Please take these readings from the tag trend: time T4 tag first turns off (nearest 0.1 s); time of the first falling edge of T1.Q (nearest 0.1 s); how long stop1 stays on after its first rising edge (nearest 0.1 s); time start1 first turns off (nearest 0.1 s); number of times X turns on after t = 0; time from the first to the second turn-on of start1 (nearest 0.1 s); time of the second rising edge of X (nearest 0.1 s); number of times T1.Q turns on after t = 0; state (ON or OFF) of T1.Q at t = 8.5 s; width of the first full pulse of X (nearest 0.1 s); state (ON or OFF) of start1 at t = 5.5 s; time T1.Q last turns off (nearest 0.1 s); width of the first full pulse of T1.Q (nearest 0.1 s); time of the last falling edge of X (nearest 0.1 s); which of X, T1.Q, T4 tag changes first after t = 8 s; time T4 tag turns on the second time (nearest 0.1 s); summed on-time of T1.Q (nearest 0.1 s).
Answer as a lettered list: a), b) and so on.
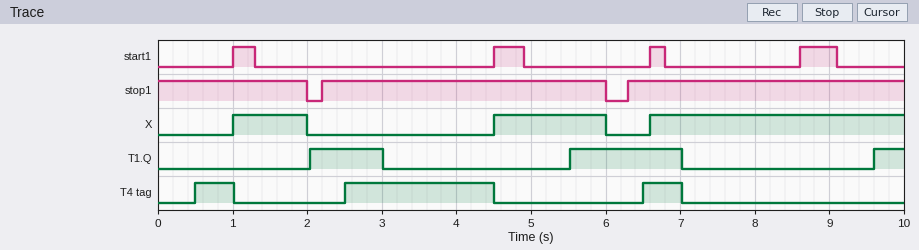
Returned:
a) 1.0 s
b) 3.0 s
c) 3.8 s
d) 1.3 s
e) 3
f) 3.5 s
g) 4.5 s
h) 3
i) OFF
j) 1.0 s
k) OFF
l) 7.0 s
m) 1.0 s
n) 6.0 s
o) T1.Q
p) 2.5 s
q) 2.9 s
